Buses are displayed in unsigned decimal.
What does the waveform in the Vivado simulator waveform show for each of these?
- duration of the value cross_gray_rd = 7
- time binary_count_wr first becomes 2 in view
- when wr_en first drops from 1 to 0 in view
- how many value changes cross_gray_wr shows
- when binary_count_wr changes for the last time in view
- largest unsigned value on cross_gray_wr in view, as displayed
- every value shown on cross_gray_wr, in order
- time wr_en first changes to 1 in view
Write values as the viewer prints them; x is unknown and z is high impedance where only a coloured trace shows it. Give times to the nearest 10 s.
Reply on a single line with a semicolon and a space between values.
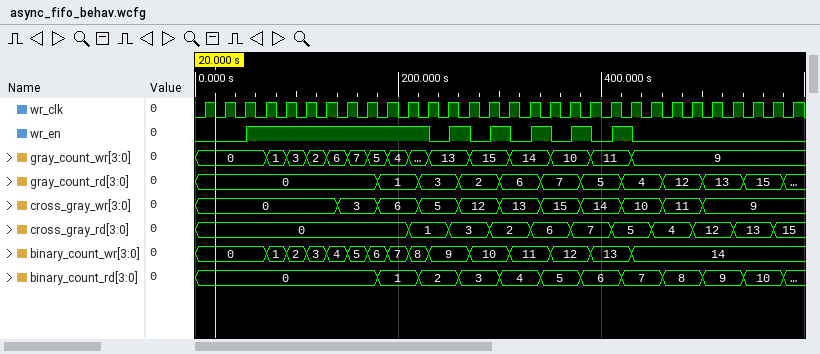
40 s; 90 s; 230 s; 10; 430 s; 15; 0, 3, 6, 5, 12, 13, 15, 14, 10, 11, 9; 50 s
